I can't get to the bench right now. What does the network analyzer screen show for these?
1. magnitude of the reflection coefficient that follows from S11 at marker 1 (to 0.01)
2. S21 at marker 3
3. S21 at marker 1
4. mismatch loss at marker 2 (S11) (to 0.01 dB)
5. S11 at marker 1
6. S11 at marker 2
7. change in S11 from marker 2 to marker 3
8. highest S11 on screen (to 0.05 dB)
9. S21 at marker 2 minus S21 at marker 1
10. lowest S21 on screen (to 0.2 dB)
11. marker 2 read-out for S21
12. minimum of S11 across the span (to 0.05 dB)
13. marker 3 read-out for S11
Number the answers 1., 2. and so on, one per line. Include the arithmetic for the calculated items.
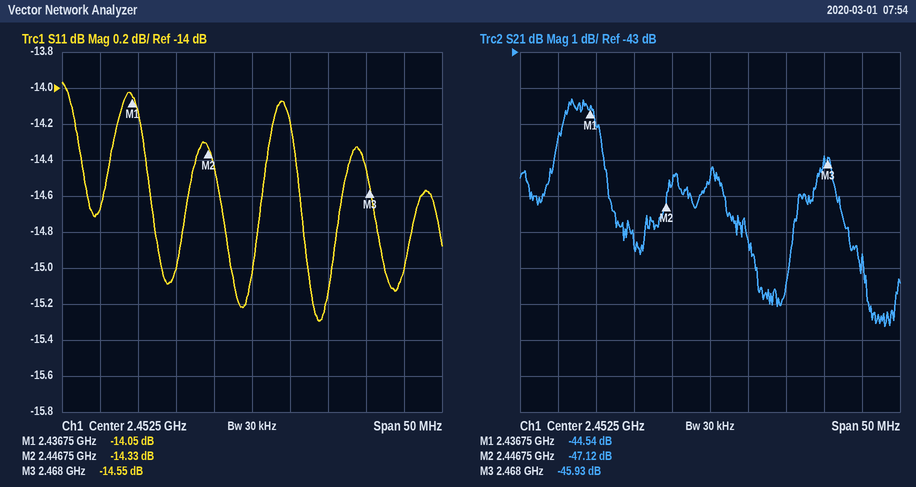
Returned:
1. 10^(-14.05/20) ≈ 0.20
2. -45.93 dB
3. -44.54 dB
4. −10 log10(1 − 10^(-14.33/10)) ≈ 0.16 dB
5. -14.05 dB
6. -14.33 dB
7. -14.55 − (-14.33) = -0.22 dB
8. -13.95 dB
9. -47.12 − (-44.54) = -2.58 dB
10. -50.6 dB
11. -47.12 dB
12. -15.30 dB
13. -14.55 dB
